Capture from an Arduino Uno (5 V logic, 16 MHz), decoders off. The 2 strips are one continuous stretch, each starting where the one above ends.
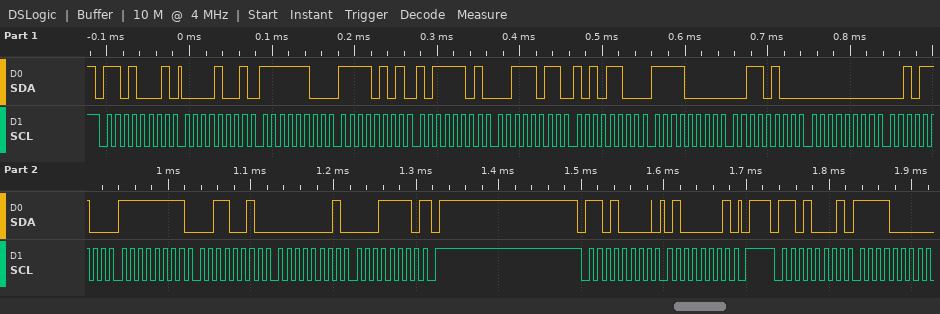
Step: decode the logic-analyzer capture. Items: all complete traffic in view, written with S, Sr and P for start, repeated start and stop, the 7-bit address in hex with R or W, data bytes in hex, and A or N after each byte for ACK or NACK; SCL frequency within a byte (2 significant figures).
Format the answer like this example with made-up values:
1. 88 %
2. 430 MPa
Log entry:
1. S 68R A 09 A FC A F5 A BD A 3B A AC A F0 A 34 A 00 A 2C A FF A 32 A 01 A 1E N P S 68W A 41 A P S 68R A F0 A
2. 100 kHz
